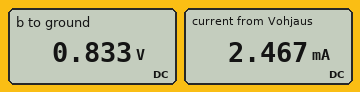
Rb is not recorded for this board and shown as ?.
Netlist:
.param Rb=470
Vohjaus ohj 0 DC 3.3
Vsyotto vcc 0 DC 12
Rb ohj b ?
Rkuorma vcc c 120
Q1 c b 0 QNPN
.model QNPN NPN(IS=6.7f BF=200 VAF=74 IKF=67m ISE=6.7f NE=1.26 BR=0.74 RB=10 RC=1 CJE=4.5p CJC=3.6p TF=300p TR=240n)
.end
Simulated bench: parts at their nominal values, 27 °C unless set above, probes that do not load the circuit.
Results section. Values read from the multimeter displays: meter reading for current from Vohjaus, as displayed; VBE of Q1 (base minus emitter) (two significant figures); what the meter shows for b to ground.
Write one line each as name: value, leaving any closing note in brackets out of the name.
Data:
meter reading for current from Vohjaus, as displayed: 2.467 mA
VBE of Q1 (base minus emitter): 830 mV
what the meter shows for b to ground: 0.833 V
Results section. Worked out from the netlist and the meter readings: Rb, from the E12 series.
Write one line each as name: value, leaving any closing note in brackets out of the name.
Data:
Rb, from the E12 series: 1 kΩ
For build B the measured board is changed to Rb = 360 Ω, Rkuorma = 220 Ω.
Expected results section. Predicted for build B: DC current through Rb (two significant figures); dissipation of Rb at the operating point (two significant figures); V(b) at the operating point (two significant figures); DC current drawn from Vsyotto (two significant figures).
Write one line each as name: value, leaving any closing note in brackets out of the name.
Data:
DC current through Rb: 6.8 mA
dissipation of Rb at the operating point: 17 mW
V(b) at the operating point: 860 mV
DC current drawn from Vsyotto: 54 mA
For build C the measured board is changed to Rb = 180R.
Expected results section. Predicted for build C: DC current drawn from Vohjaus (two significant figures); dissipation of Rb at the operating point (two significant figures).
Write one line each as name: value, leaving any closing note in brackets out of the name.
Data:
DC current drawn from Vohjaus: 13 mA
dissipation of Rb at the operating point: 31 mW
